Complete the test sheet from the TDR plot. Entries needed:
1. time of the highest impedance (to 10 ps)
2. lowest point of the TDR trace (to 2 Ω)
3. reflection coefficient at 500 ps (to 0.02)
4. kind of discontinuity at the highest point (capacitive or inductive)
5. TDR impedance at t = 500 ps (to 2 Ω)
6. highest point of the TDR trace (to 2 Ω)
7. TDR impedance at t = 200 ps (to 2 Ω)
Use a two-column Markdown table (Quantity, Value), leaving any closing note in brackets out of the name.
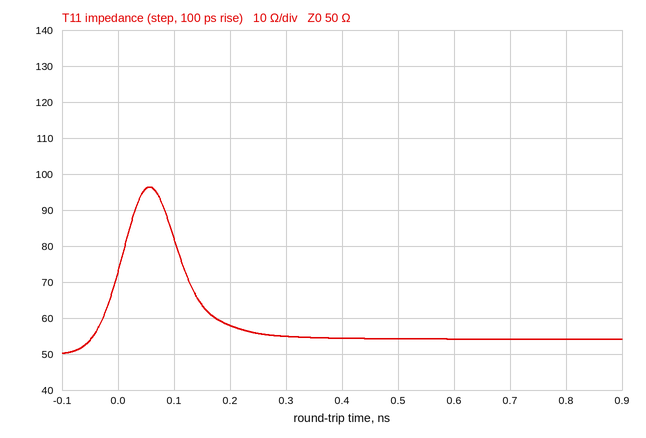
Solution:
| Quantity | Value |
|---|---|
| time of the highest impedance | 60 ps |
| lowest point of the TDR trace | 50 Ω |
| reflection coefficient at 500 ps | +0.04 |
| kind of discontinuity at the highest point | inductive |
| TDR impedance at t = 500 ps | 54 Ω |
| highest point of the TDR trace | 96 Ω |
| TDR impedance at t = 200 ps | 58 Ω |
